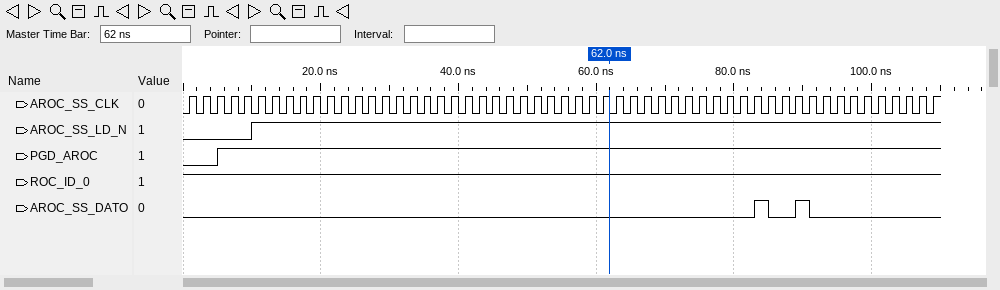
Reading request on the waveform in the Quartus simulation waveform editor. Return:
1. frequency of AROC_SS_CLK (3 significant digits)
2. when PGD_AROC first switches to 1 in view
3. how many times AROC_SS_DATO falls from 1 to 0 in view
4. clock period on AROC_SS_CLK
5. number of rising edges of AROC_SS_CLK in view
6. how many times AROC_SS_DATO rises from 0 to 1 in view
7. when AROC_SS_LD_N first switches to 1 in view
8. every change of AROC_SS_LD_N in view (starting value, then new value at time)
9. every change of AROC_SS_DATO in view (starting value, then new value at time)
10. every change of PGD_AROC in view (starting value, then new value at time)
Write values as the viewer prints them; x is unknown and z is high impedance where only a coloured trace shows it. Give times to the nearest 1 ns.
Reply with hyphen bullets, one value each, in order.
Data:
- 500 MHz
- 5 ns
- 2
- 2 ns
- 55
- 2
- 10 ns
- 0, 1 at 10 ns
- 0, 1 at 83 ns, 0 at 85 ns, 1 at 89 ns, 0 at 91 ns
- 0, 1 at 5 ns
